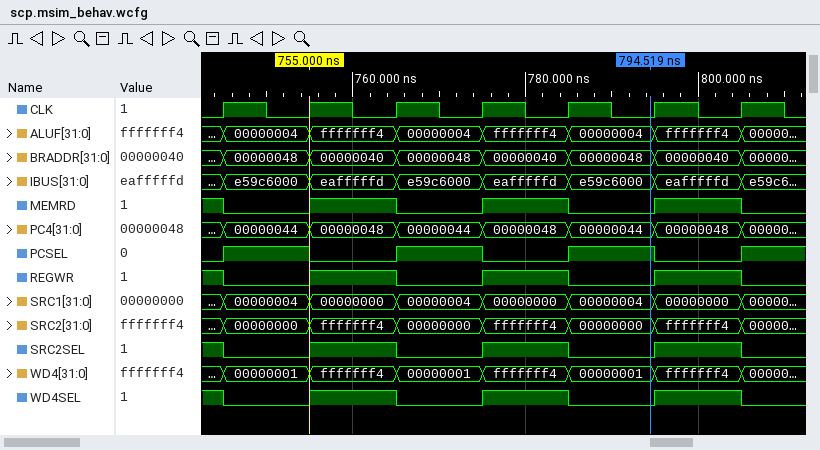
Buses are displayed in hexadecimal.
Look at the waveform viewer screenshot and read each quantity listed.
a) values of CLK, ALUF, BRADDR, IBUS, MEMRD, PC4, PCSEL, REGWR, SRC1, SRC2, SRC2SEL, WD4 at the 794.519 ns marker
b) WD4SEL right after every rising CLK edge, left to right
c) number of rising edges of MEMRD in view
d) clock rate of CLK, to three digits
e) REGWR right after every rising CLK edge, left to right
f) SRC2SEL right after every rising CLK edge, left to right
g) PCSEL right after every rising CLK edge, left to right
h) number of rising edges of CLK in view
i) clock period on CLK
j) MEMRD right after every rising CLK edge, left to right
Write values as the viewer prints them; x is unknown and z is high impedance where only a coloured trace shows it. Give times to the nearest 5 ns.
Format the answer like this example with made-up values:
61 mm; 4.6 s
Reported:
CLK=0, ALUF=00000004, BRADDR=00000048, IBUS=e59c6000, MEMRD=0, PC4=00000044, PCSEL=1, REGWR=0, SRC1=00000004, SRC2=00000000, SRC2SEL=0, WD4=00000001; 0 1 0 1 0 1 0; 3; 100 MHz; 0 1 0 1 0 1 0; 0 1 0 1 0 1 0; 1 0 1 0 1 0 1; 7; 10 ns; 0 1 0 1 0 1 0
